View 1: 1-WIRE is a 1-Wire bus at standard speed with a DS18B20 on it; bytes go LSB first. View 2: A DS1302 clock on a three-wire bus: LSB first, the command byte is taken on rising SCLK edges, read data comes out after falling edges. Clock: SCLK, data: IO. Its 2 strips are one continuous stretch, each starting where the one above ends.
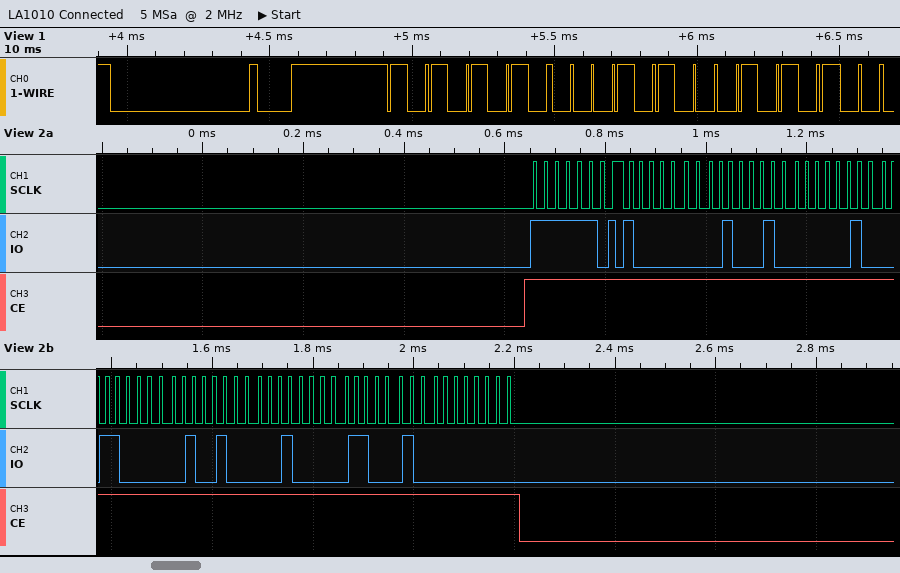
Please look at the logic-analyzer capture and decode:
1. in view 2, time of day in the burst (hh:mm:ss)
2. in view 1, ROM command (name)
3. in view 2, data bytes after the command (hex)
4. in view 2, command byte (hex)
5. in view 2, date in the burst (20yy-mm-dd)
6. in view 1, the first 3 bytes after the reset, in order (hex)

20:22:01
Match ROM
01 22 20 06 12 04 23 00
0xBF
2023-12-06
55 28 2A
